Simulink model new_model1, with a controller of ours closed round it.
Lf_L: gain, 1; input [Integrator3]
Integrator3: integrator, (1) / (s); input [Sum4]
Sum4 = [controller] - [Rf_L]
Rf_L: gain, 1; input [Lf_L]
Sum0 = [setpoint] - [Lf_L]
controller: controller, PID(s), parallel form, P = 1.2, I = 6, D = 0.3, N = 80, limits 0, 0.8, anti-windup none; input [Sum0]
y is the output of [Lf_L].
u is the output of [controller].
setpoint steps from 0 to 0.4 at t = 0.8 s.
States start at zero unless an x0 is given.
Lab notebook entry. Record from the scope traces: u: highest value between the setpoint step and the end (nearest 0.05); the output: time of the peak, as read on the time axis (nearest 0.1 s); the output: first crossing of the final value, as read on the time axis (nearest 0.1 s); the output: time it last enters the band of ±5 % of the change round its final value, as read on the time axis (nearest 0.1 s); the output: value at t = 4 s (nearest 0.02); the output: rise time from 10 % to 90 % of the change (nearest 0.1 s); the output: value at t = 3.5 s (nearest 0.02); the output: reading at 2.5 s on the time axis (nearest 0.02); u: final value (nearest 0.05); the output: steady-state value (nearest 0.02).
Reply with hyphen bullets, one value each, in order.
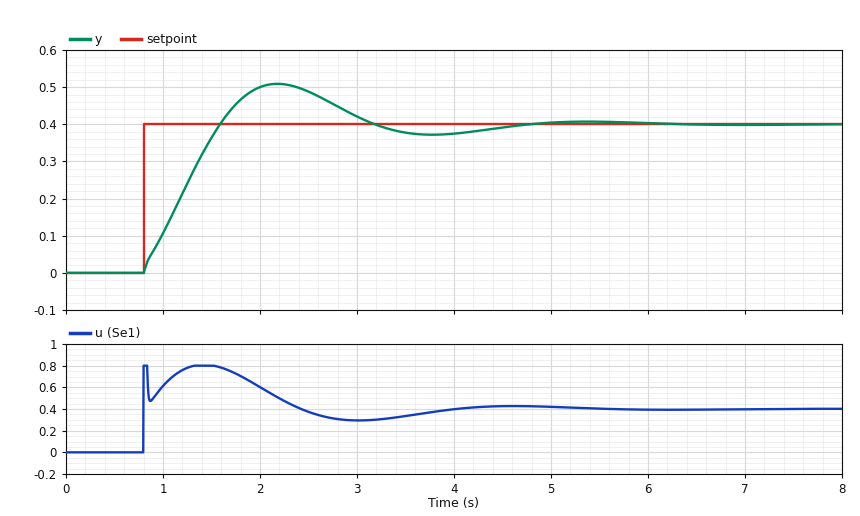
- 0.80
- 2.2 s
- 1.6 s
- 4.2 s
- 0.38
- 0.6 s
- 0.38
- 0.48
- 0.40
- 0.40
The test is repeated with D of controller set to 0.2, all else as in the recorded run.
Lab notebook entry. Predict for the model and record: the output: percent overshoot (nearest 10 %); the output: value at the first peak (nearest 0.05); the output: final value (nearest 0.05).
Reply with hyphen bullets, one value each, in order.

- 30 %
- 0.50
- 0.40
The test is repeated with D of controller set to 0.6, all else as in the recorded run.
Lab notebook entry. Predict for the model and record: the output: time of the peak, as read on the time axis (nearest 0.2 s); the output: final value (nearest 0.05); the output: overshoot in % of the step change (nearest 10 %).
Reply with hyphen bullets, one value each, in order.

- 2.4 s
- 0.40
- 30 %
